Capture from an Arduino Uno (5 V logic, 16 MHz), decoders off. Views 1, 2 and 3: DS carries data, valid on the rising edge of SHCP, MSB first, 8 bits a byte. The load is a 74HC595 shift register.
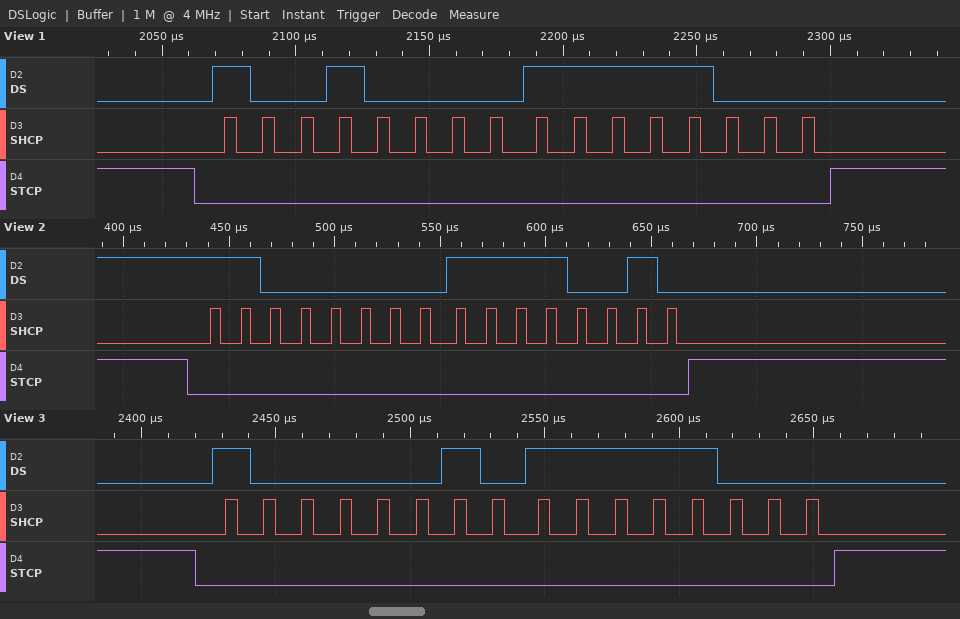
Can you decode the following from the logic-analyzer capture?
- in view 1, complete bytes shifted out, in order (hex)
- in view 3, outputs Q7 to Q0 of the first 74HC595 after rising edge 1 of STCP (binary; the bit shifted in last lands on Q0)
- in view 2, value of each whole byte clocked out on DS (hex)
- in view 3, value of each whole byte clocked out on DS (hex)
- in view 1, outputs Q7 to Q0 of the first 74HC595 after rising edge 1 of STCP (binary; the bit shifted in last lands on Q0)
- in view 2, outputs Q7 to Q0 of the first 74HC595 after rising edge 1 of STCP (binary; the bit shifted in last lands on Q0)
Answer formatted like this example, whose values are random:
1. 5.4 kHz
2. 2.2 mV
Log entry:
1. 0x90 0xF8
2. 11111000
3. C0 F2
4. 0x82 0xF8
5. 11111000
6. 11110010
